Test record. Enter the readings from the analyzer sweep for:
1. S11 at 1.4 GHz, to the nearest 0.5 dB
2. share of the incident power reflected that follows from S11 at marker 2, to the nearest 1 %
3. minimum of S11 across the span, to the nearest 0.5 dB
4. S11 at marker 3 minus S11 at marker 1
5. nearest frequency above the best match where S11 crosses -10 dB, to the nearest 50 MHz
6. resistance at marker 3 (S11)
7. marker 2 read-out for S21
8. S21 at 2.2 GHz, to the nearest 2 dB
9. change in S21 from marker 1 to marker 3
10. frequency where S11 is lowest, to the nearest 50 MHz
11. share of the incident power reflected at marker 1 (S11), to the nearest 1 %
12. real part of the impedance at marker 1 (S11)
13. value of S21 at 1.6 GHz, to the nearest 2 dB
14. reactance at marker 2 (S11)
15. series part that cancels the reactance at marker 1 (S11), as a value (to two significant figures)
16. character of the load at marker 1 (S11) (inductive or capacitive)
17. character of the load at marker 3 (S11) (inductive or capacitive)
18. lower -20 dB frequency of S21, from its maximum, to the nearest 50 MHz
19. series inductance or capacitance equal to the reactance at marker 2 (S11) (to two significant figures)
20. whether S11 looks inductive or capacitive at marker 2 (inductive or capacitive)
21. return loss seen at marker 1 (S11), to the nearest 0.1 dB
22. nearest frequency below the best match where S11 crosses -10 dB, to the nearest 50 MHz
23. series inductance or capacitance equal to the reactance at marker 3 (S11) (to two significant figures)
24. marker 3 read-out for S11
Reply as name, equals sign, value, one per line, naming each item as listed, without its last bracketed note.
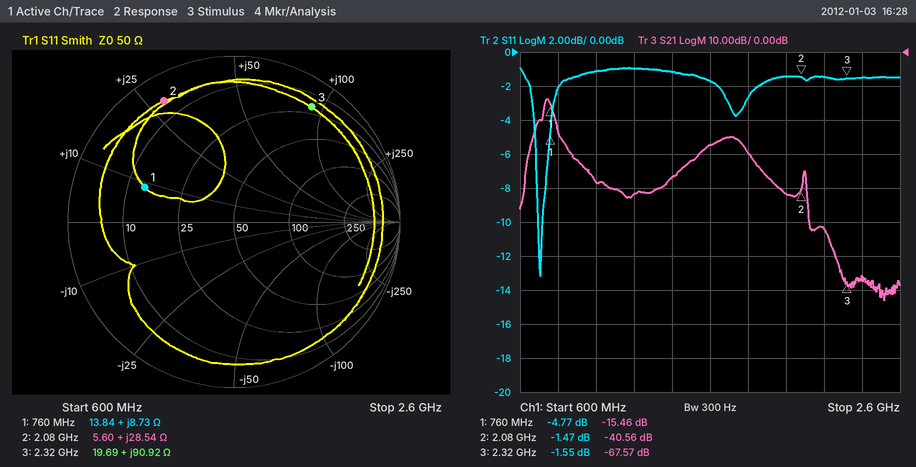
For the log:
S11 at 1.4 GHz, to the nearest 0.5 dB = -1.0 dB
share of the incident power reflected that follows from S11 at marker 2, to the nearest 1 % = 71 %
minimum of S11 across the span, to the nearest 0.5 dB = -13.0 dB
S11 at marker 3 minus S11 at marker 1 = 3.22 dB
nearest frequency above the best match where S11 crosses -10 dB, to the nearest 50 MHz = 700 MHz
resistance at marker 3 = 19.69 Ω
marker 2 read-out for S21 = -40.56 dB
S21 at 2.2 GHz, to the nearest 2 dB = -52 dB
change in S21 from marker 1 to marker 3 = -52.11 dB
frequency where S11 is lowest, to the nearest 50 MHz = 700 MHz
share of the incident power reflected at marker 1 (S11), to the nearest 1 % = 33 %
real part of the impedance at marker 1 = 13.84 Ω
value of S21 at 1.6 GHz, to the nearest 2 dB = -28 dB
reactance at marker 2 = +28.54 Ω
series part that cancels the reactance at marker 1 (S11), as a value = 24 pF
character of the load at marker 1 (S11) = inductive
character of the load at marker 3 (S11) = inductive
lower -20 dB frequency of S21, from its maximum, to the nearest 50 MHz = 650 MHz
series inductance or capacitance equal to the reactance at marker 2 (S11) = 2.2 nH
whether S11 looks inductive or capacitive at marker 2 = inductive
return loss seen at marker 1 (S11), to the nearest 0.1 dB = 4.8 dB
nearest frequency below the best match where S11 crosses -10 dB, to the nearest 50 MHz = 700 MHz
series inductance or capacitance equal to the reactance at marker 3 (S11) = 6.2 nH
marker 3 read-out for S11 = -1.55 dB
